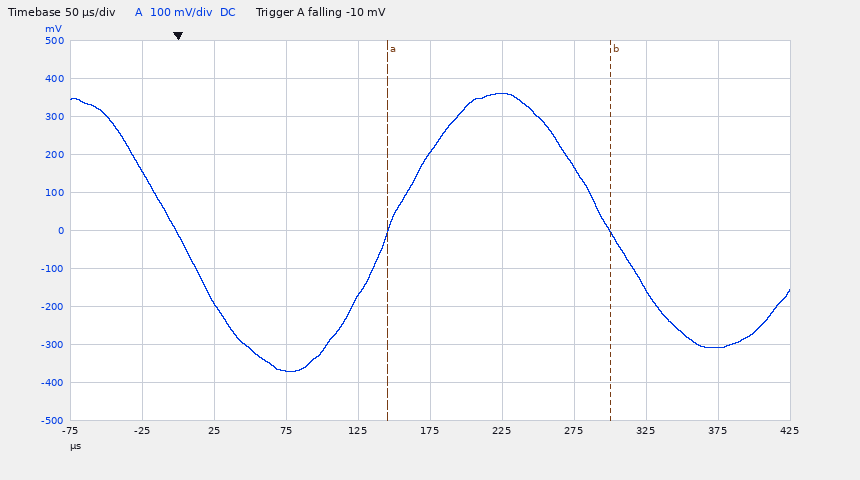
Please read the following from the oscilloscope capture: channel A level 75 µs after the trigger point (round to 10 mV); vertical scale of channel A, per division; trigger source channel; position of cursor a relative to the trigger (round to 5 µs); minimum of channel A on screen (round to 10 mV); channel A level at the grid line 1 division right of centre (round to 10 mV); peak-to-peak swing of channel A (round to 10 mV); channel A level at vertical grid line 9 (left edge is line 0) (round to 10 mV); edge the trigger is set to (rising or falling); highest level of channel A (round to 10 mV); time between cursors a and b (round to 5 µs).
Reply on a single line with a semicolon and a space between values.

-370 mV; 100 mV; channel A; +145 µs; -370 mV; 360 mV; 730 mV; -310 mV; falling; 360 mV; 155 µs
